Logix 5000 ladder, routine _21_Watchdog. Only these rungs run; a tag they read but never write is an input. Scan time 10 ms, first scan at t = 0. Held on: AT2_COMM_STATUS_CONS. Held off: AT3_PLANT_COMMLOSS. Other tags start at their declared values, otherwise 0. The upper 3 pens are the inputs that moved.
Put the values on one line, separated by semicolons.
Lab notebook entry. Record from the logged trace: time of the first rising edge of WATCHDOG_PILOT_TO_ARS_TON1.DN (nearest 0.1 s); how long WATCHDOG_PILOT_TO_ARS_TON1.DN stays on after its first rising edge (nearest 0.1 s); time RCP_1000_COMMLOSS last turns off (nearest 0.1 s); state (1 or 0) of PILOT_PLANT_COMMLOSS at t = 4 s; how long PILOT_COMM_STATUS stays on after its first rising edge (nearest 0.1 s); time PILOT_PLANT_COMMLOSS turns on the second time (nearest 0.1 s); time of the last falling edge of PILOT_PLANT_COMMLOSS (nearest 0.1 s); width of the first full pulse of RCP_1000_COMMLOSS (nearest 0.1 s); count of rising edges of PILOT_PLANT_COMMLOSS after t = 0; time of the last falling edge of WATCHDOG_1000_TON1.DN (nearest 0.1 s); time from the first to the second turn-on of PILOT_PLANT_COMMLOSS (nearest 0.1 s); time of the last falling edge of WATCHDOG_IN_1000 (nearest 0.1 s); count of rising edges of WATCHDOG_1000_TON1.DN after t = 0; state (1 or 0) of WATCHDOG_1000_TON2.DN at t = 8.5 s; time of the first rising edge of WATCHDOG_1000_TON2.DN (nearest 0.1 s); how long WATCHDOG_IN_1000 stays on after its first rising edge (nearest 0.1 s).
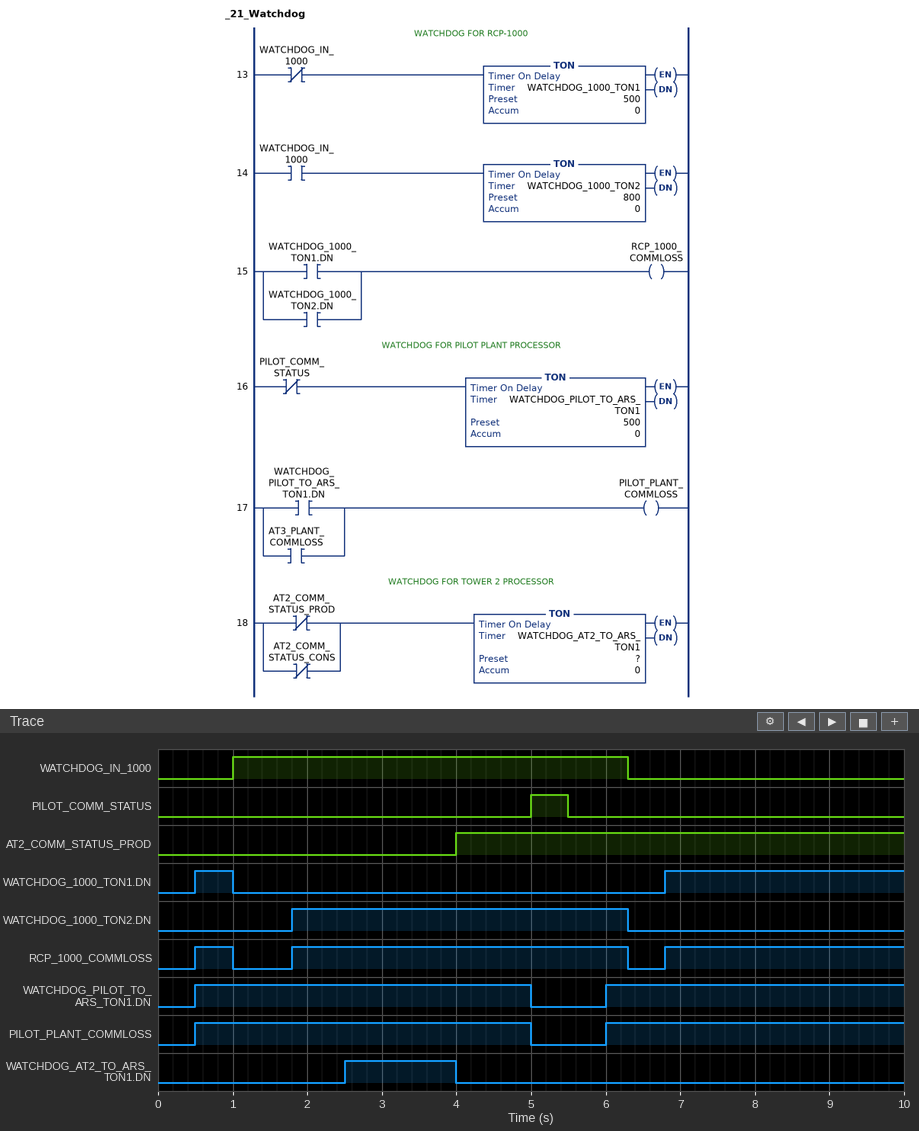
0.5 s; 4.5 s; 6.3 s; 1; 0.5 s; 6.0 s; 5.0 s; 0.5 s; 2; 1.0 s; 5.5 s; 6.3 s; 2; 0; 1.8 s; 5.3 s
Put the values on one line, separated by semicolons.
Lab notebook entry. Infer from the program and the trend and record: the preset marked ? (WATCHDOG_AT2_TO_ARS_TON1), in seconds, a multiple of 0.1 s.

2.5 s
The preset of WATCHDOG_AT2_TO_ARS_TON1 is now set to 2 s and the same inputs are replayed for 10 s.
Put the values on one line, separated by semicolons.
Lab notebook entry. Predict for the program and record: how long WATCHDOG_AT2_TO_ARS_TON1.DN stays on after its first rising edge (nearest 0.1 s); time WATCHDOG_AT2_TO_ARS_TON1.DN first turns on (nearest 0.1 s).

2.0 s; 2.0 s
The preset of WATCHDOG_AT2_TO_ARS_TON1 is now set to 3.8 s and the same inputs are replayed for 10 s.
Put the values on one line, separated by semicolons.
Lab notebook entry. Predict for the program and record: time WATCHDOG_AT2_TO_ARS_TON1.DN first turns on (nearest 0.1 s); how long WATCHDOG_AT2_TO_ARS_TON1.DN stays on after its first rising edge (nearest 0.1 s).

3.8 s; 0.2 s
